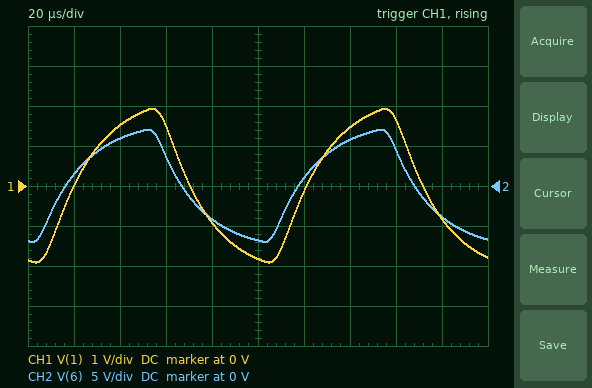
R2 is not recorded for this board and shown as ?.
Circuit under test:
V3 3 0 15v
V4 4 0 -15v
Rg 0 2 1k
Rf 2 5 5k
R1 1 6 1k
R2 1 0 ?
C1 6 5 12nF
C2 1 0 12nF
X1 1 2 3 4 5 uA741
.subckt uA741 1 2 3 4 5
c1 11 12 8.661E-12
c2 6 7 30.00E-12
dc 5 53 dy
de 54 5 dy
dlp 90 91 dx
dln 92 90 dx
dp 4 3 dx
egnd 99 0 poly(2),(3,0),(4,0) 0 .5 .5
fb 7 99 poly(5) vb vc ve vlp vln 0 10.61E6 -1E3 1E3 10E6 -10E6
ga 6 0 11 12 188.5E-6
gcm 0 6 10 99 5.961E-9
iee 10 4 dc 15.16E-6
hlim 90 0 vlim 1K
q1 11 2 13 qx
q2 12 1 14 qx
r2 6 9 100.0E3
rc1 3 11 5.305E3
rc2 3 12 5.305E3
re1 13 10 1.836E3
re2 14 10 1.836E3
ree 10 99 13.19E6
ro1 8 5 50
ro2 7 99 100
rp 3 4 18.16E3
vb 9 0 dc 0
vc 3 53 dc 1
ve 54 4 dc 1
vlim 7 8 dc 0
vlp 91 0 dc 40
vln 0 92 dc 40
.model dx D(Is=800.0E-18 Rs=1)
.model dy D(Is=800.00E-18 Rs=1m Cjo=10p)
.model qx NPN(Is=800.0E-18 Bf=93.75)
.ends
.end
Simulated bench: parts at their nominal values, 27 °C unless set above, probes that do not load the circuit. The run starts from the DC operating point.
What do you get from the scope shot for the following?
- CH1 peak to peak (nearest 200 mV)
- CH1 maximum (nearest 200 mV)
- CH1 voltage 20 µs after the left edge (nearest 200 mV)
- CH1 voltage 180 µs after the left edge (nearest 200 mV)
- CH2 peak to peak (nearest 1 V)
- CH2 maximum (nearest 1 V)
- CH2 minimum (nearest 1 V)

3.8 V
2.0 V
0 V
-800 mV
14 V
7 V
-7 V
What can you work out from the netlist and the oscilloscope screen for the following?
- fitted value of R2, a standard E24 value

390 Ω
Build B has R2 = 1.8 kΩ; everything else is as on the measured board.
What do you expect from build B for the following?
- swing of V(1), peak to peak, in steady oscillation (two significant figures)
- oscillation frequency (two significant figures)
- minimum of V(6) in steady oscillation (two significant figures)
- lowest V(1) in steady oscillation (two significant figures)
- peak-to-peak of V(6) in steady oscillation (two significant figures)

13 V
4.1 kHz
-11 V
-6.5 V
22 V
